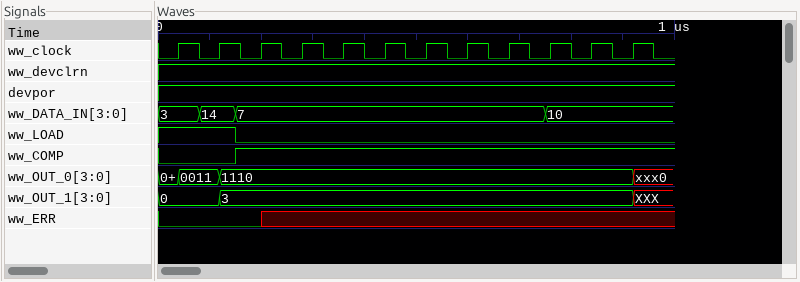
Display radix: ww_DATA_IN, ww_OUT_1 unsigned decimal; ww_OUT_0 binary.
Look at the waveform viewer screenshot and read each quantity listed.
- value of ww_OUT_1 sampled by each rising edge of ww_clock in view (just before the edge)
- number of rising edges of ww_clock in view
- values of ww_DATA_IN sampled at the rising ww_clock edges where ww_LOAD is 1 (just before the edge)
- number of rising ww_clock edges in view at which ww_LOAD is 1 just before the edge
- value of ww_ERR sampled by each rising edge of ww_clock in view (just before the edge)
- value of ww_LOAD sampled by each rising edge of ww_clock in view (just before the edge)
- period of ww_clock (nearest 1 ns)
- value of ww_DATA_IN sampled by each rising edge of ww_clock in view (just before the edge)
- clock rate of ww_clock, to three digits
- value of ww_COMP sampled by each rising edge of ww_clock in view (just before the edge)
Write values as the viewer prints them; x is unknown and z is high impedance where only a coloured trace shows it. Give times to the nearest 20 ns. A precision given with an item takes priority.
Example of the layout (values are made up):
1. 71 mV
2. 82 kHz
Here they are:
1. 0, 0, 3, 3, 3, 3, 3, 3, 3, 3, 3, 3
2. 12
3. 3, 14
4. 2
5. 0 0 0 x x x x x x x x x
6. 1 1 0 0 0 0 0 0 0 0 0 0
7. 80 ns
8. 3, 14, 7, 7, 7, 7, 7, 7, 7, 10, 10, 10
9. 12.5 MHz
10. 0 0 1 1 1 1 1 1 1 1 1 1
